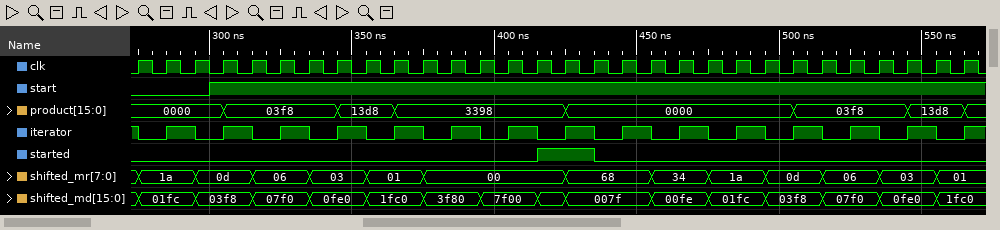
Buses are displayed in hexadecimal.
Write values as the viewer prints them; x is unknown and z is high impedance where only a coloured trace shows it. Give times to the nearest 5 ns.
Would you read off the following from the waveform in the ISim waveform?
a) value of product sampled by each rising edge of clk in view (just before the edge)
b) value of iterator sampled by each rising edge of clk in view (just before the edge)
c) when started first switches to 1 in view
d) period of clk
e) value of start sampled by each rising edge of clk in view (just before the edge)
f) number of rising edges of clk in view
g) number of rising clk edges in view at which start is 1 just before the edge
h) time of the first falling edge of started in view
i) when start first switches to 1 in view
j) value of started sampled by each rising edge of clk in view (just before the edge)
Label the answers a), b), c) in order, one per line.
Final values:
a) 0000, 0000, 0000, 0000, 03f8, 03f8, 03f8, 03f8, 13d8, 13d8, 3398, 3398, 3398, 3398, 3398, 3398, 0000, 0000, 0000, 0000, 0000, 0000, 0000, 0000, 03f8, 03f8, 03f8, 03f8, 13d8, 13d8
b) 1 0 1 0 1 0 1 0 1 0 1 0 1 0 1 0 1 0 1 0 1 0 1 0 1 0 1 0 1 0
c) 415 ns
d) 10 ns
e) 0 0 0 1 1 1 1 1 1 1 1 1 1 1 1 1 1 1 1 1 1 1 1 1 1 1 1 1 1 1
f) 30
g) 27
h) 435 ns
i) 300 ns
j) 0 0 0 0 0 0 0 0 0 0 0 0 0 0 0 1 1 0 0 0 0 0 0 0 0 0 0 0 0 0
